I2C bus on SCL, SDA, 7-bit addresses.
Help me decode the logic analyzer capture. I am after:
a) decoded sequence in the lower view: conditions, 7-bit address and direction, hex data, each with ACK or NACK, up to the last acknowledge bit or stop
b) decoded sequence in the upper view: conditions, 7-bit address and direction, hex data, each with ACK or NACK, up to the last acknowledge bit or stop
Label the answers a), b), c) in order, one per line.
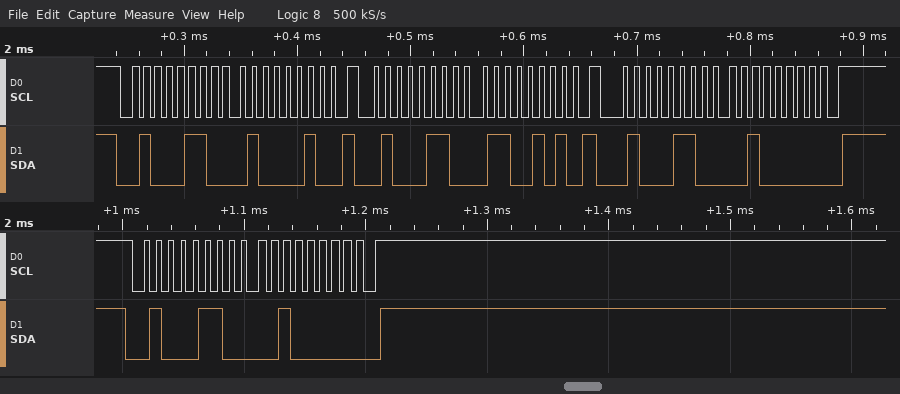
a) start, address 23 write ACK, 20 ACK, stop
b) start, address 23 write ACK, 42 ACK, repeated start, address 23 write ACK, 65 ACK, repeated start, address 23 write ACK, 20 ACK, stop
